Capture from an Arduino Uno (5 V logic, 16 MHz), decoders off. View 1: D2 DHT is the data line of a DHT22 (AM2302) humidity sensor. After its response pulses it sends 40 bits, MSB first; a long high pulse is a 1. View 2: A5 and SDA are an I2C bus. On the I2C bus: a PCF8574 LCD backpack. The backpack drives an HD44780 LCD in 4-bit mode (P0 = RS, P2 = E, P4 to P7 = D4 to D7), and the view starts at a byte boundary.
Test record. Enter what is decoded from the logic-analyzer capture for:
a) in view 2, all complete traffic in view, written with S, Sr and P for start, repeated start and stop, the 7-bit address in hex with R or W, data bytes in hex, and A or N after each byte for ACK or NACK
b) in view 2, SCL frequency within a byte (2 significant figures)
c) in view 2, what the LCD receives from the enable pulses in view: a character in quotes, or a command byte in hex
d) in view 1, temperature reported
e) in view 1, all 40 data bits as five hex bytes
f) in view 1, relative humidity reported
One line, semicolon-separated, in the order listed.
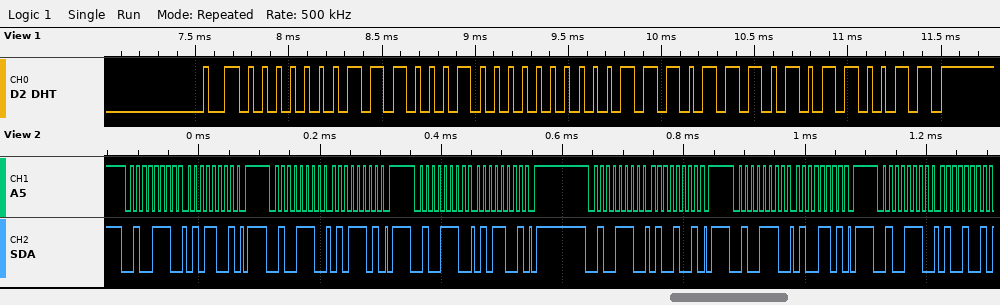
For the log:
S 27W A 59 A P S 27W A 5D A P S 27W A 59 A P S 27W A 49 A P S 27W A 4D A P S 27W A 49 A; 100 kHz; 'T'; 23.8 °C; 01 C4 00 EE B3; 45.2 %
